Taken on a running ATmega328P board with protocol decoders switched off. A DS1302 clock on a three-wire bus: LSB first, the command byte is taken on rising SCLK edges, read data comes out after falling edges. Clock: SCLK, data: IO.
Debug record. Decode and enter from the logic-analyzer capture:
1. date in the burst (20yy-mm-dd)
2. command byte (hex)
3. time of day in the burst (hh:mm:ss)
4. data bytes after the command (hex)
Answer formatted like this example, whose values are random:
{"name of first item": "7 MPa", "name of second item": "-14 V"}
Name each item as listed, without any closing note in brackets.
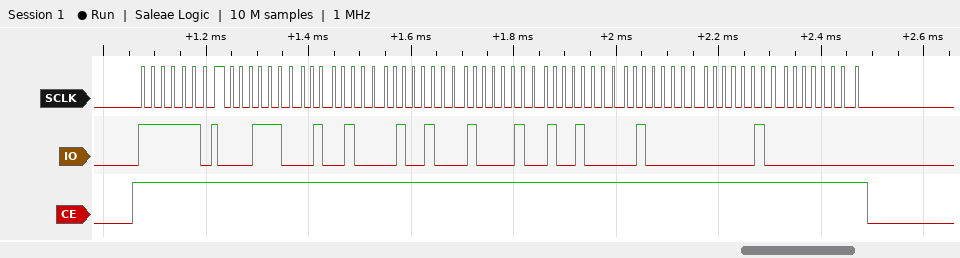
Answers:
{"date in the burst": "2020-09-21", "command byte": "0xBF", "time of day in the burst": "12:12:38", "data bytes after the command": "38 12 12 21 09 02 20 00"}
